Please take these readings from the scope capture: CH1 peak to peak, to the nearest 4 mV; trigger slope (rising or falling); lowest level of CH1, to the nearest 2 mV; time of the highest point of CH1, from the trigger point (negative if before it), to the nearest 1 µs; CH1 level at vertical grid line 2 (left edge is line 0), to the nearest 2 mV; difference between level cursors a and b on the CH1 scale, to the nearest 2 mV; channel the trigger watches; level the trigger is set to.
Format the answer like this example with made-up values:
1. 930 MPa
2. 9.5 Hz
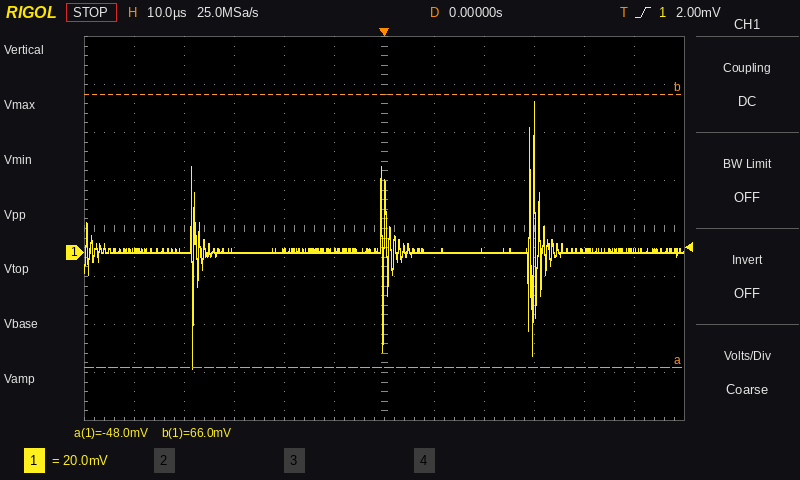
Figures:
1. 112 mV
2. rising
3. -48 mV
4. +30 µs
5. 0 mV
6. 114 mV
7. CH1
8. 2.00 mV
